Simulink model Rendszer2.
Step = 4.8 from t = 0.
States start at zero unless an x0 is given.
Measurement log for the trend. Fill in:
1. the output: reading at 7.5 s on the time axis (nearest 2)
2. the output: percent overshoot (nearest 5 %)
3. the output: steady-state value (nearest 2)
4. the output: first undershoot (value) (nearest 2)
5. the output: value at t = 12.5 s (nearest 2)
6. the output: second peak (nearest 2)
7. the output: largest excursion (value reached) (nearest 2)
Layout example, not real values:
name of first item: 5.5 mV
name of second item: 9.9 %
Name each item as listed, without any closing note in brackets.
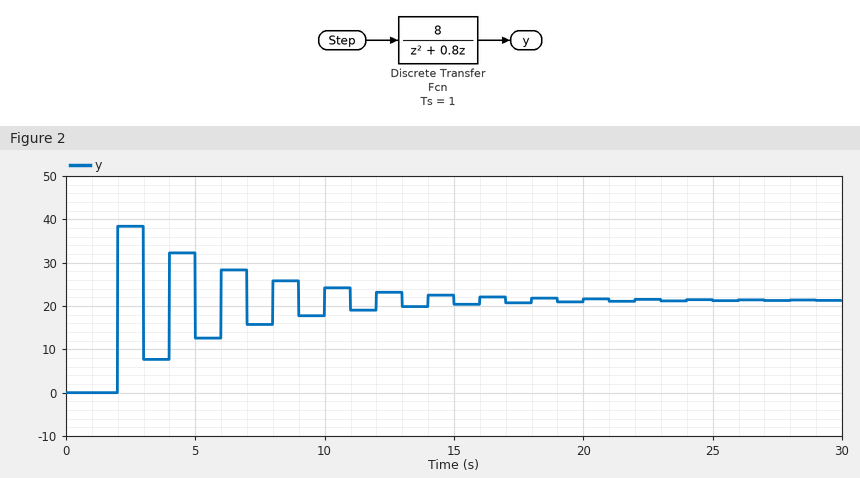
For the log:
the output: reading at 7.5 s on the time axis: 16
the output: percent overshoot: 80 %
the output: steady-state value: 22
the output: first undershoot (value): 8
the output: value at t = 12.5 s: 24
the output: second peak: 32
the output: largest excursion (value reached): 38
